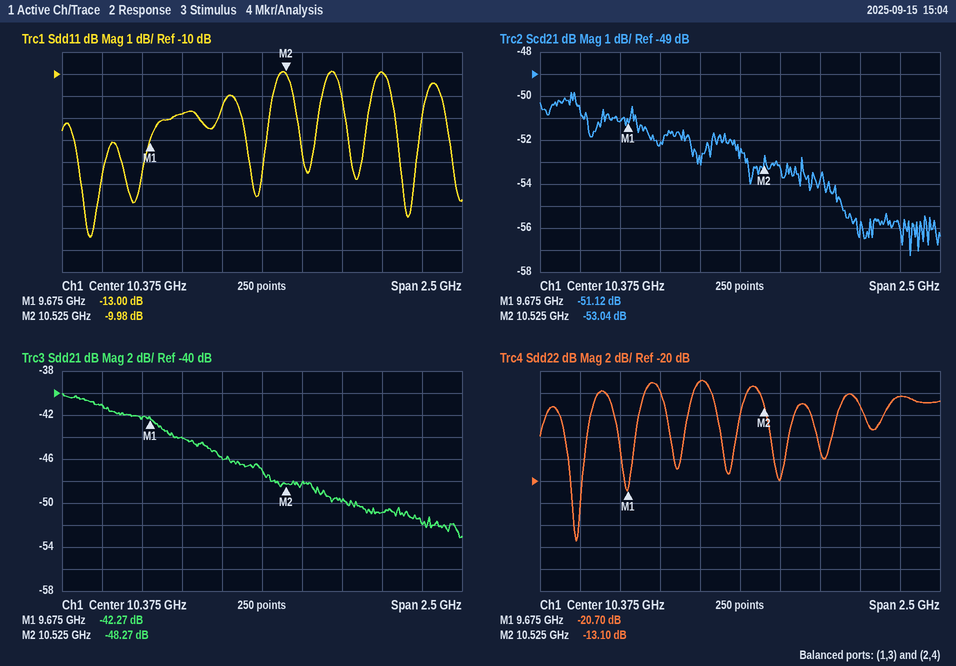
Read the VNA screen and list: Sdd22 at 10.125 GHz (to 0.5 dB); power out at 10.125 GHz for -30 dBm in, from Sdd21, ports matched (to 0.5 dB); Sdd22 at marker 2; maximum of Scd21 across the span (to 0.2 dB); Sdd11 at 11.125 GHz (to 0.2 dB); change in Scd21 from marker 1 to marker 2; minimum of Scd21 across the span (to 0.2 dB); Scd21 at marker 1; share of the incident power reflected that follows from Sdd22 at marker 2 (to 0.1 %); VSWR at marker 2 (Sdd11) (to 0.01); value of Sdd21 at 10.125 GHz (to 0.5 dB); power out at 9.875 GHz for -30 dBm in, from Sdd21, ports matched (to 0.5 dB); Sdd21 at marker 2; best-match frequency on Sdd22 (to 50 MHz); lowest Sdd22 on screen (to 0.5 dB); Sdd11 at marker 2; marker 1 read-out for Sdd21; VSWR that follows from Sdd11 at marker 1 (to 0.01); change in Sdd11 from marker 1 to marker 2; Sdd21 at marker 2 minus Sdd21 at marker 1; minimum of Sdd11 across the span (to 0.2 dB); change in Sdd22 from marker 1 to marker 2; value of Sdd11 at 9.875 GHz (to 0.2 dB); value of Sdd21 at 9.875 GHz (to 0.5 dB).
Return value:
-11.0 dB
-76.0 dBm
-13.10 dB
-49.8 dB
-10.0 dB
-1.92 dB
-57.2 dB
-51.12 dB
4.9 %
1.93
-46.0 dB
-74.0 dBm
-48.27 dB
9.35 GHz
-25.5 dB
-9.98 dB
-42.27 dB
1.58
3.02 dB
-6.00 dB
-17.4 dB
7.60 dB
-11.8 dB
-44.0 dB
